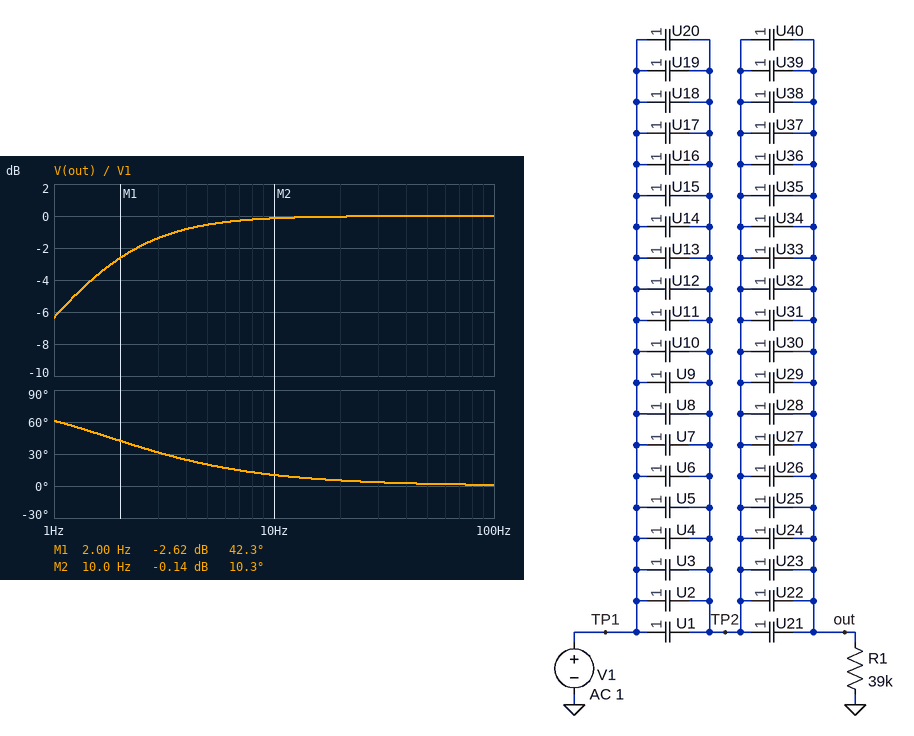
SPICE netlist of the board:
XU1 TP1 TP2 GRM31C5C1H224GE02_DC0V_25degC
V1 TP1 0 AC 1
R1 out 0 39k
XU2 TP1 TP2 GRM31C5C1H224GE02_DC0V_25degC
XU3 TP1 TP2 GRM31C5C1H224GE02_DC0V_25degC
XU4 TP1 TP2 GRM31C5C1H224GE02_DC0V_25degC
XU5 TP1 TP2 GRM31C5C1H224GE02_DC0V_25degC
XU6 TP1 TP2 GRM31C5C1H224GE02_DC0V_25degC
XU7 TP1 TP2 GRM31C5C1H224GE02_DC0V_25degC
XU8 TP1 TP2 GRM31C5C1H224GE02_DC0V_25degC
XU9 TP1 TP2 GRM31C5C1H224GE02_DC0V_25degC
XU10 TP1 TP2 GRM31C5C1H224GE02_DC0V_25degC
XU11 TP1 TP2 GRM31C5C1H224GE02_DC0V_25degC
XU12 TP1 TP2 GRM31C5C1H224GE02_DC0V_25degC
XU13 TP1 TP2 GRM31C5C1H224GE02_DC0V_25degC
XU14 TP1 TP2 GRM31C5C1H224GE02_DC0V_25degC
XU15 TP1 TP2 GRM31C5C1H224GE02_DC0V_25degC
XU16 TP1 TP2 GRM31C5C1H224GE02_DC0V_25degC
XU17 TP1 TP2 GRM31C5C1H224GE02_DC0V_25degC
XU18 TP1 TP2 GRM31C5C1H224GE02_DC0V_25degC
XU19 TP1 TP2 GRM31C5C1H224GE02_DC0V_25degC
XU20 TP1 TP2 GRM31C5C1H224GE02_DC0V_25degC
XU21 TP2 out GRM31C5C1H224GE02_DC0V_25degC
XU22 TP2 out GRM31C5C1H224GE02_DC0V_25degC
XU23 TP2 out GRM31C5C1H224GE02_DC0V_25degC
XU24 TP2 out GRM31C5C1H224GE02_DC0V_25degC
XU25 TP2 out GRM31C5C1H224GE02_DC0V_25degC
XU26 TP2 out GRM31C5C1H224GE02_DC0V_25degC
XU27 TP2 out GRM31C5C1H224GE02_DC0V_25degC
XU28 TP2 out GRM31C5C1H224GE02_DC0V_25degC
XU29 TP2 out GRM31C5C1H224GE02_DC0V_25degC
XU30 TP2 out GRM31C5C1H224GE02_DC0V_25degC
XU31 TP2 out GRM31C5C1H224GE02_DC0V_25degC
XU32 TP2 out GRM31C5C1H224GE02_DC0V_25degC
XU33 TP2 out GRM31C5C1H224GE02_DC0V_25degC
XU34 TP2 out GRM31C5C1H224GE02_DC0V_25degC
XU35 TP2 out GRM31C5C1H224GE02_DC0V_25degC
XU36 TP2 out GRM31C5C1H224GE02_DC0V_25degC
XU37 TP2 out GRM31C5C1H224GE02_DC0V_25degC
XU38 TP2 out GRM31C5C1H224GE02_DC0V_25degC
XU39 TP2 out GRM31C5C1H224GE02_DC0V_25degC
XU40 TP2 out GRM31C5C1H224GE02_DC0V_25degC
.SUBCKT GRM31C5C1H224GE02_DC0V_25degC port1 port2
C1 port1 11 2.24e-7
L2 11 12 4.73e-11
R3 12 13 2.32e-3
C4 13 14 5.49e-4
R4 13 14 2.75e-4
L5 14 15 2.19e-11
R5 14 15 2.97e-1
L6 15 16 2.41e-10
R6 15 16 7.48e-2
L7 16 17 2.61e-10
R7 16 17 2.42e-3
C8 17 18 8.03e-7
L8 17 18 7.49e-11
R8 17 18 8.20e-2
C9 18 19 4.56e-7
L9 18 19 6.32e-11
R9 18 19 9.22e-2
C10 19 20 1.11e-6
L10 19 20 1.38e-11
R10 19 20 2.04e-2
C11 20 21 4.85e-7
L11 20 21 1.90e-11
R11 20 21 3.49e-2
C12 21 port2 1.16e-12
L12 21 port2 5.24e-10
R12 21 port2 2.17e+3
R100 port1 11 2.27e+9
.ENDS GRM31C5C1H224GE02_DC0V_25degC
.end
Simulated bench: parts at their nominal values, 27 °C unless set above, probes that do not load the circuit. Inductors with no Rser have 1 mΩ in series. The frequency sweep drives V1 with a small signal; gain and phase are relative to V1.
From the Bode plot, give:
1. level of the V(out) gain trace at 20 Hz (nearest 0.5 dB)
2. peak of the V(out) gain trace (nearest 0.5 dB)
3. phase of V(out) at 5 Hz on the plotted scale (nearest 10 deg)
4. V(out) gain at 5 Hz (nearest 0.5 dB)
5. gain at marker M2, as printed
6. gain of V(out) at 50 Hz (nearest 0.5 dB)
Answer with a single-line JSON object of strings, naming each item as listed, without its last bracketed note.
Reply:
{"level of the V(out) gain trace at 20 Hz": "0 dB", "peak of the V(out) gain trace": "0 dB", "phase of V(out) at 5 Hz on the plotted scale": "20 deg", "V(out) gain at 5 Hz": "-0.5 dB", "gain at marker M2, as printed": "-0.14 dB", "gain of V(out) at 50 Hz": "0 dB"}
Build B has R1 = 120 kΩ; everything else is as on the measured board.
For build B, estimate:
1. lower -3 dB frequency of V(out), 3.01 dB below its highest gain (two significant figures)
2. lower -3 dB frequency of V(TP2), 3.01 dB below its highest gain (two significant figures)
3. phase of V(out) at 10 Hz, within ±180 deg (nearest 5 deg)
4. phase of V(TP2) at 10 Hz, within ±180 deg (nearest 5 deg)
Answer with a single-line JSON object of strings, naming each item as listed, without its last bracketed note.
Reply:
{"lower -3 dB frequency of V(out), 3.01 dB below its highest gain": "590 mHz", "lower -3 dB frequency of V(TP2), 3.01 dB below its highest gain": "420 mHz", "phase of V(out) at 10 Hz, within ±180 deg": "5 deg", "phase of V(TP2) at 10 Hz, within ±180 deg": "0 deg"}
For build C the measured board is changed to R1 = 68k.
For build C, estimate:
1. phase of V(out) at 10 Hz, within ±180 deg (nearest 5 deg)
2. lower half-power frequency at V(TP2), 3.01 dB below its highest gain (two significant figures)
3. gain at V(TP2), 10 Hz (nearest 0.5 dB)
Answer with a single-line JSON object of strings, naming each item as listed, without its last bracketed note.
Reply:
{"phase of V(out) at 10 Hz, within ±180 deg": "5 deg", "lower half-power frequency at V(TP2), 3.01 dB below its highest gain": "740 mHz", "gain at V(TP2), 10 Hz": "0 dB"}
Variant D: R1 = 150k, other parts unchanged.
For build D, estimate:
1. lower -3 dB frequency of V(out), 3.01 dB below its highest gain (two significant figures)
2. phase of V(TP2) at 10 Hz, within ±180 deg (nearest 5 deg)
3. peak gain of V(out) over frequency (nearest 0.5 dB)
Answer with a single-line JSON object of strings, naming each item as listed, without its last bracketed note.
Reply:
{"lower -3 dB frequency of V(out), 3.01 dB below its highest gain": "470 mHz", "phase of V(TP2) at 10 Hz, within ±180 deg": "0 deg", "peak gain of V(out) over frequency": "0 dB"}
